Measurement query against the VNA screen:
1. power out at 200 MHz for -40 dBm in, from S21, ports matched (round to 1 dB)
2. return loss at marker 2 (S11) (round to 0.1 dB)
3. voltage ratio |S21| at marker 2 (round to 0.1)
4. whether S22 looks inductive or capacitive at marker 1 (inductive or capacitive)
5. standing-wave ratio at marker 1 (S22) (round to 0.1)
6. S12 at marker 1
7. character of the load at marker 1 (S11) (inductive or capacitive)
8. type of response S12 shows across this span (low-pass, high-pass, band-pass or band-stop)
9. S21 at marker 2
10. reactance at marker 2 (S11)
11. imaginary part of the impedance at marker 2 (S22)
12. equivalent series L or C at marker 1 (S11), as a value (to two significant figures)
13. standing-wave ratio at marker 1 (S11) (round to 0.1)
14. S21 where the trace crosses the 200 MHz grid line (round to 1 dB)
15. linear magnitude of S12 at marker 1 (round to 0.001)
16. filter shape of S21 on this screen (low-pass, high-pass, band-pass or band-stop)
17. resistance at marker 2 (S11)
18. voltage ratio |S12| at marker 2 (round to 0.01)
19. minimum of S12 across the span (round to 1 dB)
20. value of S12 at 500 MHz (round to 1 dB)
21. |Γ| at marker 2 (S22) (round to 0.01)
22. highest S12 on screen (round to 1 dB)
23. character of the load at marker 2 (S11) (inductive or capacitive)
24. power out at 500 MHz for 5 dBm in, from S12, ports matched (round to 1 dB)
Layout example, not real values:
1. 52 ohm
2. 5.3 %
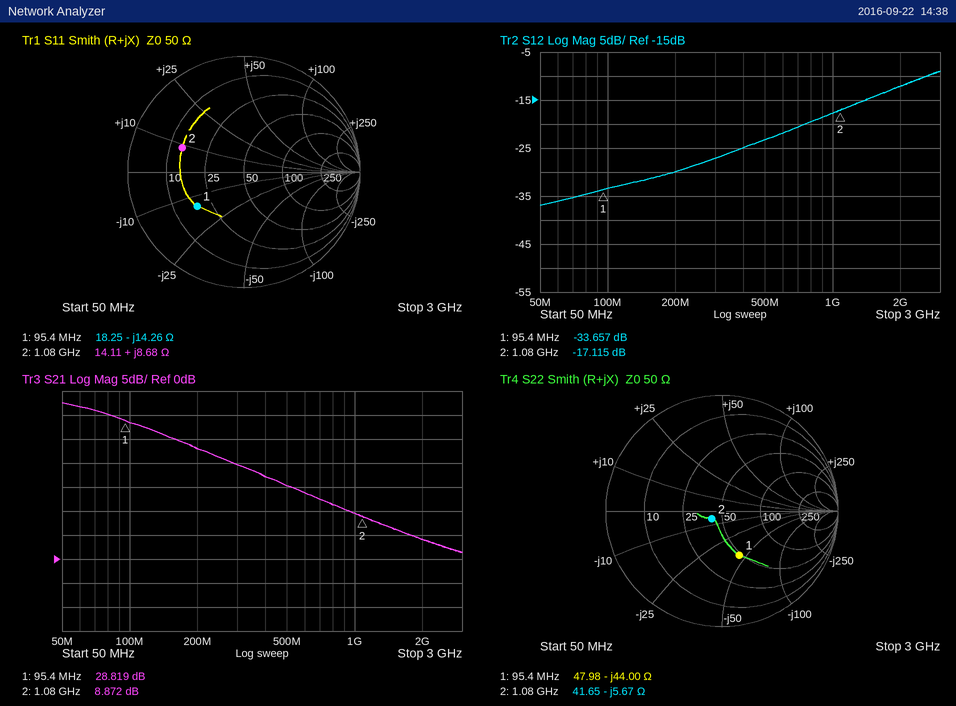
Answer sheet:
1. -17 dBm
2. 4.9 dB
3. 2.8
4. capacitive
5. 2.4
6. -33.657 dB
7. capacitive
8. high-pass
9. 8.872 dB
10. +8.68 Ω
11. -5.67 Ω
12. 120 pF
13. 3.0
14. 23 dB
15. 0.021
16. low-pass
17. 14.11 Ω
18. 0.14
19. -37 dB
20. -23 dB
21. 0.11
22. -9 dB
23. inductive
24. -18 dBm
